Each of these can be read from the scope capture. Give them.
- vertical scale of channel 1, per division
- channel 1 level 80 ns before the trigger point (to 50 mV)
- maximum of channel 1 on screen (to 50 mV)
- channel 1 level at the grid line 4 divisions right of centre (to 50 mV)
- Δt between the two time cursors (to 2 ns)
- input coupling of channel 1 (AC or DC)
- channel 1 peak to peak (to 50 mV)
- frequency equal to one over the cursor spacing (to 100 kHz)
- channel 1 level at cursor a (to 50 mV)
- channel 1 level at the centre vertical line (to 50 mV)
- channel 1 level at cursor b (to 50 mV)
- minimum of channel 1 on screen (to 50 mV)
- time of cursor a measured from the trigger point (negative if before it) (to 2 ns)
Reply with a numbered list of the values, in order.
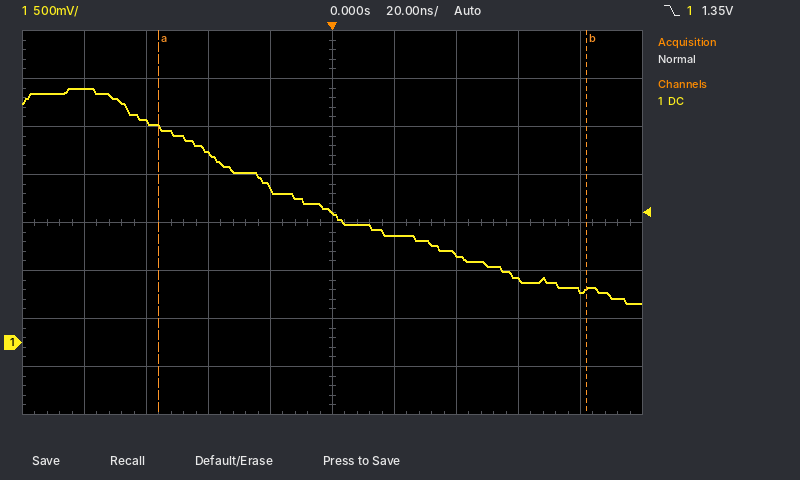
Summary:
1. 500 mV
2. 2.65 V
3. 2.65 V
4. 550 mV
5. 138 ns
6. DC
7. 2.25 V
8. 7.2 MHz
9. 2.25 V
10. 1.35 V
11. 550 mV
12. 400 mV
13. -56 ns
